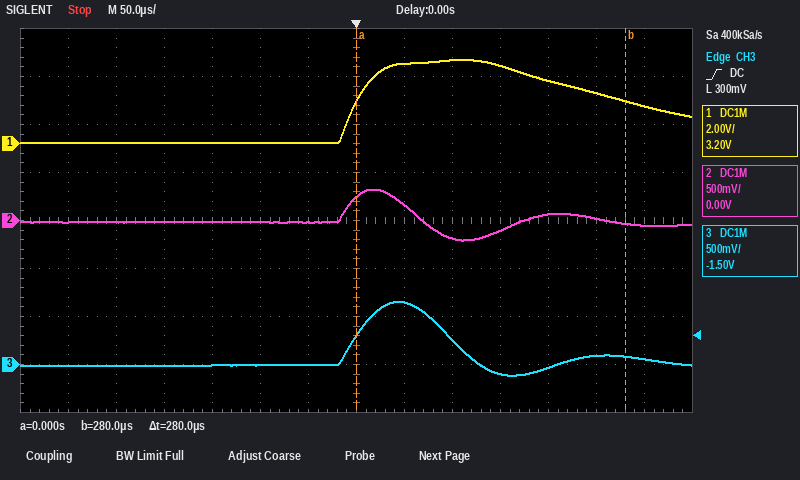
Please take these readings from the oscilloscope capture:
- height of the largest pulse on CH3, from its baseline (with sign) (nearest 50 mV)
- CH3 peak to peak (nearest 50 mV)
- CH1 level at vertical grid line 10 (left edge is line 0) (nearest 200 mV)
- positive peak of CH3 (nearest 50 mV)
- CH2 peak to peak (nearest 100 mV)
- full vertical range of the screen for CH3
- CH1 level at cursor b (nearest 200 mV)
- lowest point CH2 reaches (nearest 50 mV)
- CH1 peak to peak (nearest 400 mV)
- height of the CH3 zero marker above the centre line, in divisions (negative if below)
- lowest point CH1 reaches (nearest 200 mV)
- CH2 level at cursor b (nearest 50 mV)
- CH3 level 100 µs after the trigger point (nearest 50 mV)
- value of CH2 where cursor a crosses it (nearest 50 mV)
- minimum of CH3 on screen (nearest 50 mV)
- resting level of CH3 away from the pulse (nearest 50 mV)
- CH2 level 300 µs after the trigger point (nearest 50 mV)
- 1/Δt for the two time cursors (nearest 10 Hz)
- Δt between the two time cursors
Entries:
+650 mV
750 mV
3.2 V
650 mV
500 mV
4 V
1.8 V
-200 mV
3.6 V
-3.0 div
0.0 V
-50 mV
250 mV
250 mV
-100 mV
0 mV
-50 mV
3.57 kHz
280 µs
